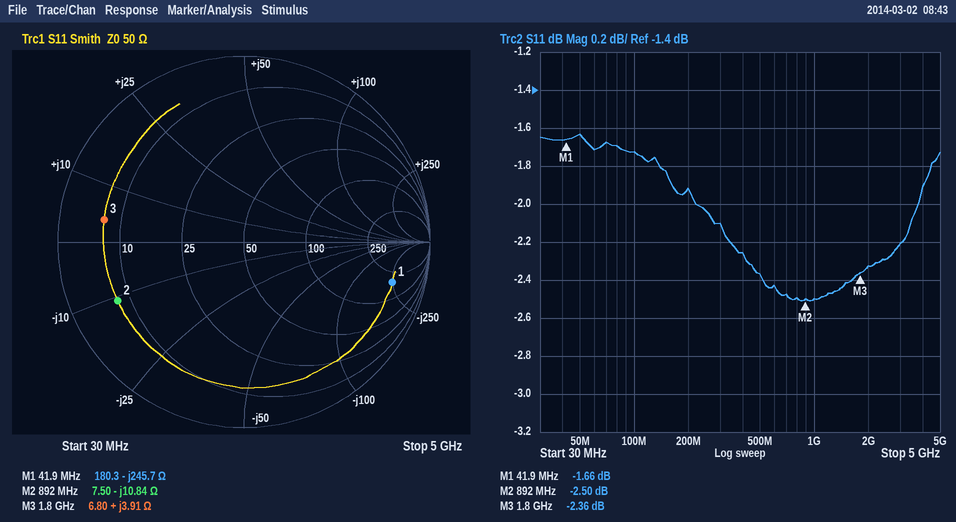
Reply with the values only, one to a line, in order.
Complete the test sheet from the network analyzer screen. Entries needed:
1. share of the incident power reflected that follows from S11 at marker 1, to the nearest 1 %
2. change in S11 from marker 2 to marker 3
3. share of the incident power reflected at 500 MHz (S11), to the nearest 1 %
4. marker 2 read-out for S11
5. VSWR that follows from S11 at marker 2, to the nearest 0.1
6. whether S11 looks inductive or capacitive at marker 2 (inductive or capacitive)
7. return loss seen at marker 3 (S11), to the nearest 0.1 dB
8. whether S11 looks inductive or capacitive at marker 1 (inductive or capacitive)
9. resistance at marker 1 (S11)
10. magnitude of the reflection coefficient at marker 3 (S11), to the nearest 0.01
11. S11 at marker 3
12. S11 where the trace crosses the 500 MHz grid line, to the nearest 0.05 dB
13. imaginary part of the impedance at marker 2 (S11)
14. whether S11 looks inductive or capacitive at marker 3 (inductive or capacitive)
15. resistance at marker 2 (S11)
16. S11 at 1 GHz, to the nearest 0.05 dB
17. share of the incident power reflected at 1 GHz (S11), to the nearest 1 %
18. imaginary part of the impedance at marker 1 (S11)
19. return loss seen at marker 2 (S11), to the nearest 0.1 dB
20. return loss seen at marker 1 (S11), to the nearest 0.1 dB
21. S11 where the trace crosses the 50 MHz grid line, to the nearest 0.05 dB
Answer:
68 %
0.14 dB
58 %
-2.50 dB
7.0
capacitive
2.4 dB
capacitive
180.3 Ω
0.76
-2.36 dB
-2.35 dB
-10.84 Ω
inductive
7.50 Ω
-2.50 dB
56 %
-245.7 Ω
2.5 dB
1.7 dB
-1.65 dB
